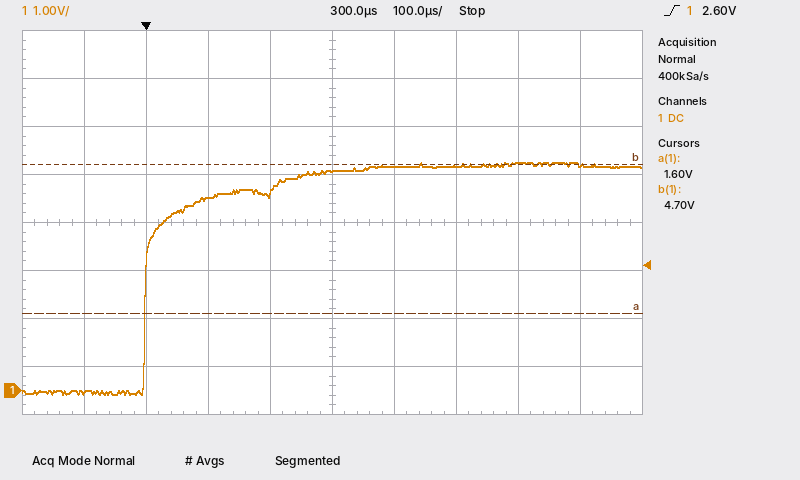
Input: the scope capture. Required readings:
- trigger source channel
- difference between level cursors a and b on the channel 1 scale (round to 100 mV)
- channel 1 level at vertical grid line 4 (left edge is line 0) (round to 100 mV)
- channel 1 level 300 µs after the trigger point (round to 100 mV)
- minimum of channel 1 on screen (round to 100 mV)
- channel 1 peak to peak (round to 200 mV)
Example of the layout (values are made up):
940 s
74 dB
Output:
channel 1
3.1 V
4.1 V
4.6 V
-100 mV
4.8 V
